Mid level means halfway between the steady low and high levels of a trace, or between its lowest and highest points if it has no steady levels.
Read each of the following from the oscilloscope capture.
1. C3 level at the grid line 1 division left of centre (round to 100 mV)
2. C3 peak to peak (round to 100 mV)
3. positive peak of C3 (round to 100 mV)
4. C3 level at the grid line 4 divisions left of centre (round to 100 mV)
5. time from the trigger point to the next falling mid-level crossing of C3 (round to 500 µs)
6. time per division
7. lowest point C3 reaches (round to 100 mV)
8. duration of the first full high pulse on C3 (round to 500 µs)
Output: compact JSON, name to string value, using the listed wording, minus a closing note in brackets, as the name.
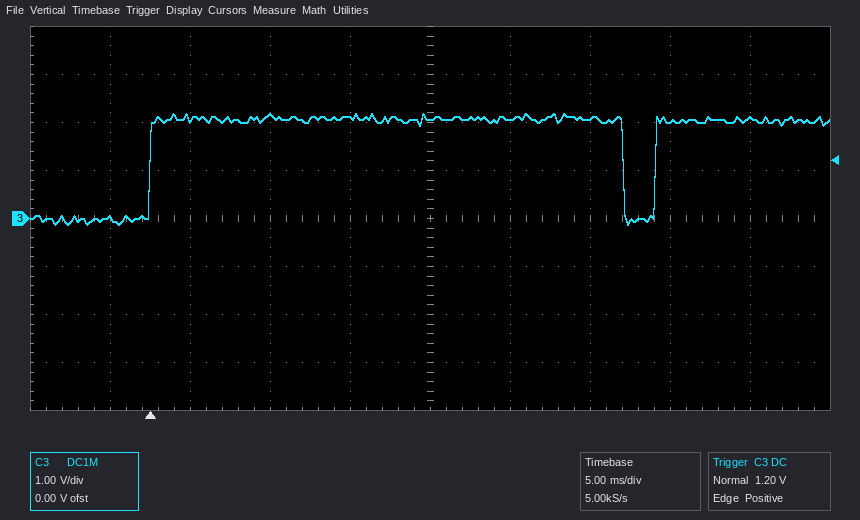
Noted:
{"C3 level at the grid line 1 division left of centre": "2.1 V", "C3 peak to peak": "2.3 V", "positive peak of C3": "2.2 V", "C3 level at the grid line 4 divisions left of centre": "0.0 V", "time from the trigger point to the next falling mid-level crossing of C3": "29.5 ms", "time per division": "5 ms", "lowest point C3 reaches": "-100 mV", "duration of the first full high pulse on C3": "29.5 ms"}
